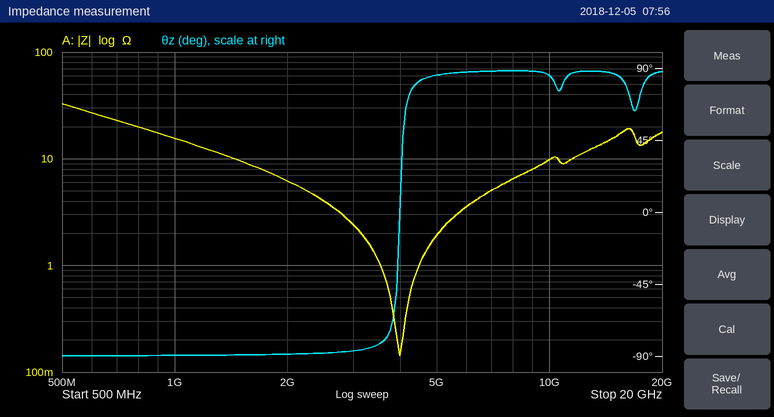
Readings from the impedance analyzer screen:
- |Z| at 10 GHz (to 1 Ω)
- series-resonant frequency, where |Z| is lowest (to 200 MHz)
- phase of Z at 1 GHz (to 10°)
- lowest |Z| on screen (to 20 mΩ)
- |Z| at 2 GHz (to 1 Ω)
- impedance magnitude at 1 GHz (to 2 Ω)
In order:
10 Ω
4.0 GHz
-90°
140 mΩ
6 Ω
16 Ω
